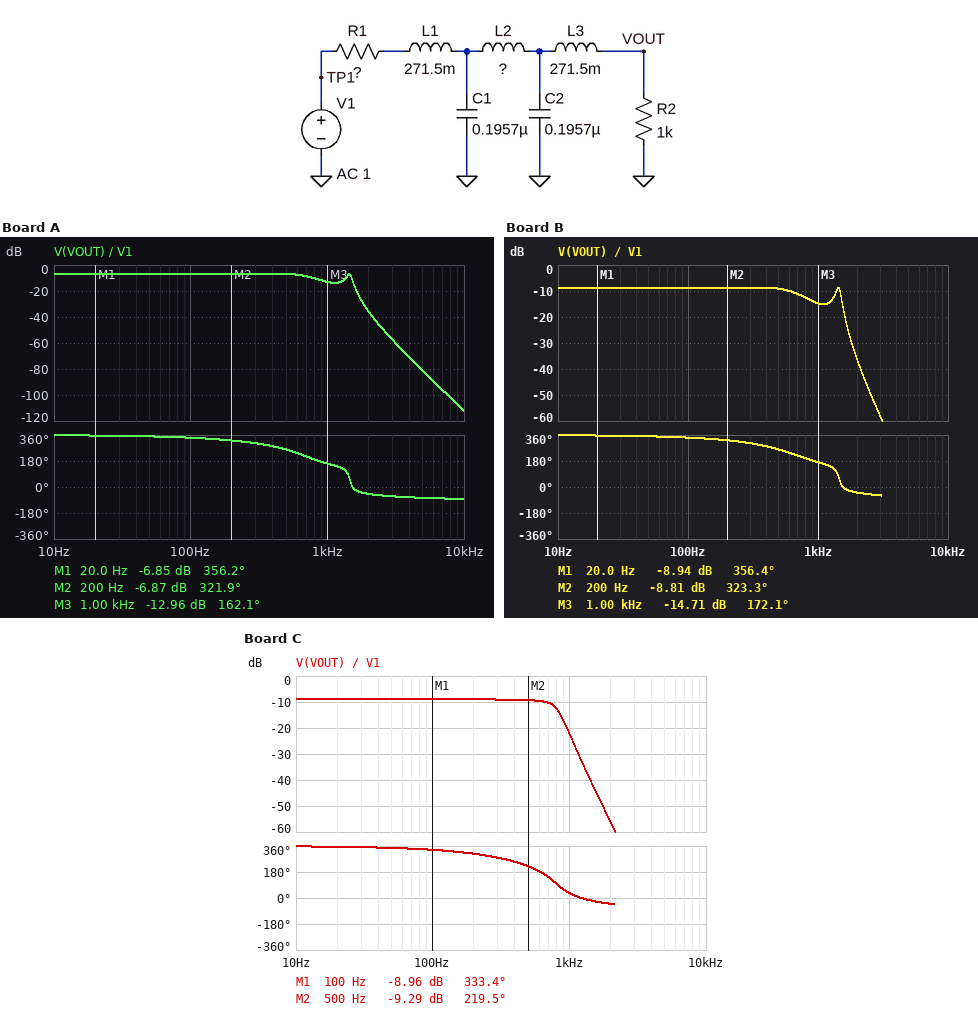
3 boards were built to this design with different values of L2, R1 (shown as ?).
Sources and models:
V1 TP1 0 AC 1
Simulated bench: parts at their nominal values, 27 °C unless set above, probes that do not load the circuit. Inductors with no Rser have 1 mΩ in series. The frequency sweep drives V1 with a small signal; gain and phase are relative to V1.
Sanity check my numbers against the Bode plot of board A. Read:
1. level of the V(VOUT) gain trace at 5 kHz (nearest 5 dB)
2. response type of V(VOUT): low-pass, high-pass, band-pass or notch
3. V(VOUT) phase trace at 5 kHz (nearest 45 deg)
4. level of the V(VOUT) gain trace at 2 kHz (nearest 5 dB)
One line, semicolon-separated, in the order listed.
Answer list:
-80 dB; low-pass; -90 deg; -35 dB
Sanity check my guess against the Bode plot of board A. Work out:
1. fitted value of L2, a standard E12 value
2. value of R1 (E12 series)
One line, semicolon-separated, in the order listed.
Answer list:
150 mH; 1.2 kΩ
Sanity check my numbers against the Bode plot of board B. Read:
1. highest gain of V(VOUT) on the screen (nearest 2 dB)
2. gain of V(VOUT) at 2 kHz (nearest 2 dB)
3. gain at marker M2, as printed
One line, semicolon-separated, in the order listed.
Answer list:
-8 dB; -36 dB; -8.81 dB
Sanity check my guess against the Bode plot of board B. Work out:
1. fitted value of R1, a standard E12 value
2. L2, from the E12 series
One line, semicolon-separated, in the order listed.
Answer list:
1.8 kΩ; 150 mH
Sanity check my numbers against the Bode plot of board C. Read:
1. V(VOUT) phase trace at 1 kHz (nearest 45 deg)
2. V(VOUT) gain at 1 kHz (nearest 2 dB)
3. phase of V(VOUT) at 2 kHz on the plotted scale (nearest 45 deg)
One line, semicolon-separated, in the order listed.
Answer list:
45 deg; -22 dB; -45 deg
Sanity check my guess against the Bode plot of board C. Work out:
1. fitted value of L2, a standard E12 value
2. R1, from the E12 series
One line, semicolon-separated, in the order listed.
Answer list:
820 mH; 1.8 kΩ
